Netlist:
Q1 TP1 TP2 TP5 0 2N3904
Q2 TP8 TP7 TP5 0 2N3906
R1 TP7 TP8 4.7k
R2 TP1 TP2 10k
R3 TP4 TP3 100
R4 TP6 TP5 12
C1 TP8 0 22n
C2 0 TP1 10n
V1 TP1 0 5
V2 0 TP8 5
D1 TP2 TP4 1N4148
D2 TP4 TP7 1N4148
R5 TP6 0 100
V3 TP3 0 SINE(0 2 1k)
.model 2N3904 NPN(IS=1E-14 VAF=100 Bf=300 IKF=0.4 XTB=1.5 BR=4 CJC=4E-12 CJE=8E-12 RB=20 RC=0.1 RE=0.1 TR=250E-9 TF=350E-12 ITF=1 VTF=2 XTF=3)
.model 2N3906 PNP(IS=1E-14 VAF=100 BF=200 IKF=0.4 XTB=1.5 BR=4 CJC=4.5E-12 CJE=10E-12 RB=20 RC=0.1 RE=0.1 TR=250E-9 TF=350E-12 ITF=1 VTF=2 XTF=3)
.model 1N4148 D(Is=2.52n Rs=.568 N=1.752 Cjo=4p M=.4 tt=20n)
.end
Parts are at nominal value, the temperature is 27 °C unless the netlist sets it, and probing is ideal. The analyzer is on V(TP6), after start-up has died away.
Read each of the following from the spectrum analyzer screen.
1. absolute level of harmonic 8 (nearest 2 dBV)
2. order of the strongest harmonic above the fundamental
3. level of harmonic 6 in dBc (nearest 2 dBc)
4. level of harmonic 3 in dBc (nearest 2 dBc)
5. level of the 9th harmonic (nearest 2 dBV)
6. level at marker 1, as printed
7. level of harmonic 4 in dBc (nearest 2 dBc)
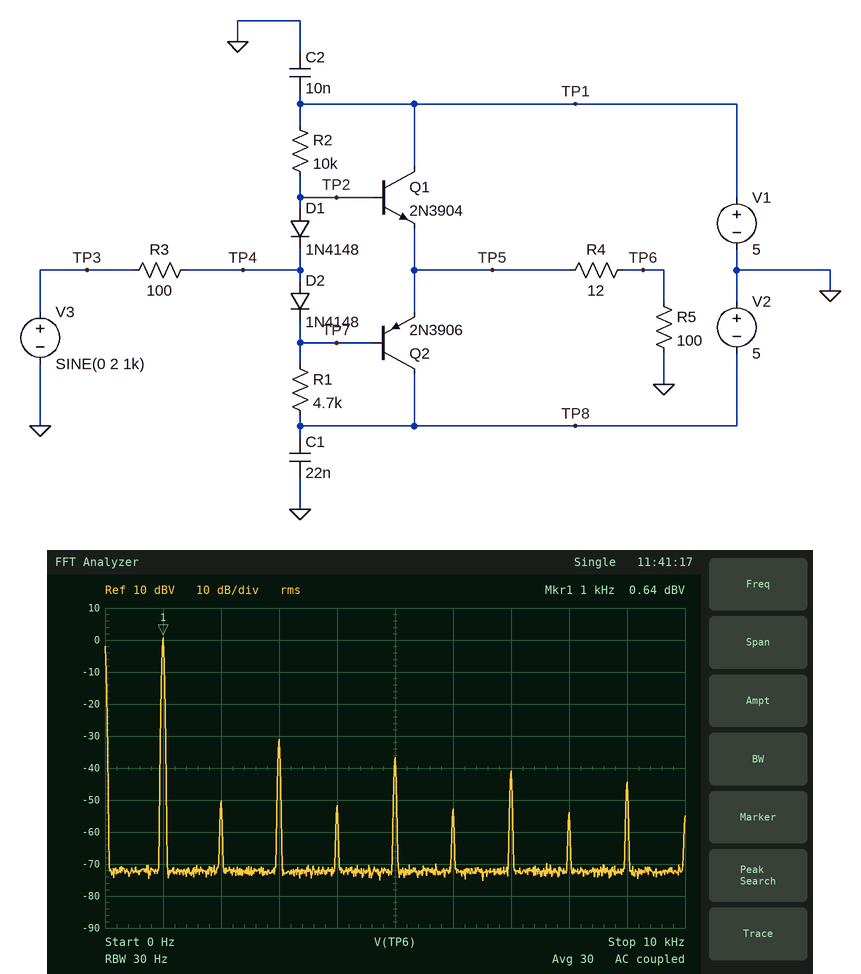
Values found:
-54 dBV
3
-54 dBc
-32 dBc
-44 dBV
0.64 dBV
-52 dBc
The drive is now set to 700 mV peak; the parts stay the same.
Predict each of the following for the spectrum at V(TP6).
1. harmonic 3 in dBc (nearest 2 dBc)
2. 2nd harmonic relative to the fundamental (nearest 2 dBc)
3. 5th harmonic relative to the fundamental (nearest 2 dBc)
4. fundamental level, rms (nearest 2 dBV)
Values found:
-24 dBc
-34 dBc
-32 dBc
-10 dBV
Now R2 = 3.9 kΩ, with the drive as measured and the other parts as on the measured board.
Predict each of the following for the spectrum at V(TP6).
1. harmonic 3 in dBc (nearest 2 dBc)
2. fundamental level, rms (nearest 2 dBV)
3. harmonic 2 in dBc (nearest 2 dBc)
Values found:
-34 dBc
0 dBV
-56 dBc
